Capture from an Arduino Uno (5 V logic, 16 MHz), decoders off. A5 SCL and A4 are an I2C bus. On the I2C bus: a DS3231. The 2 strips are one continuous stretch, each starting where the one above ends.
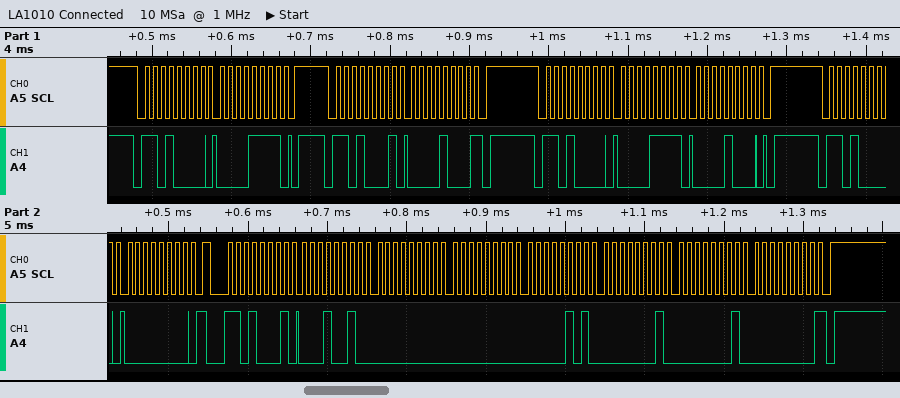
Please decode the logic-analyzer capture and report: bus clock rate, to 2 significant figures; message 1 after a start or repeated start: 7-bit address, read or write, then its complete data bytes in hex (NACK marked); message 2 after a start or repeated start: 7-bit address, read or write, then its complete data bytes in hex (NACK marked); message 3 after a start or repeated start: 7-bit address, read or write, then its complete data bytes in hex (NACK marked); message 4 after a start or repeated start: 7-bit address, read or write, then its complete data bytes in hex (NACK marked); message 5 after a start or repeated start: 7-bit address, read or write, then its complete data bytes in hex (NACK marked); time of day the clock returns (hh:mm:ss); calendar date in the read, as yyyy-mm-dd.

100 kHz
0x68 write: 0F
0x68 read: 08 NACK
0x68 write: 0F 08
0x68 write: 00
0x68 read: 12 00 00 05 01 01 00 NACK
00:00:12
2000-01-01
